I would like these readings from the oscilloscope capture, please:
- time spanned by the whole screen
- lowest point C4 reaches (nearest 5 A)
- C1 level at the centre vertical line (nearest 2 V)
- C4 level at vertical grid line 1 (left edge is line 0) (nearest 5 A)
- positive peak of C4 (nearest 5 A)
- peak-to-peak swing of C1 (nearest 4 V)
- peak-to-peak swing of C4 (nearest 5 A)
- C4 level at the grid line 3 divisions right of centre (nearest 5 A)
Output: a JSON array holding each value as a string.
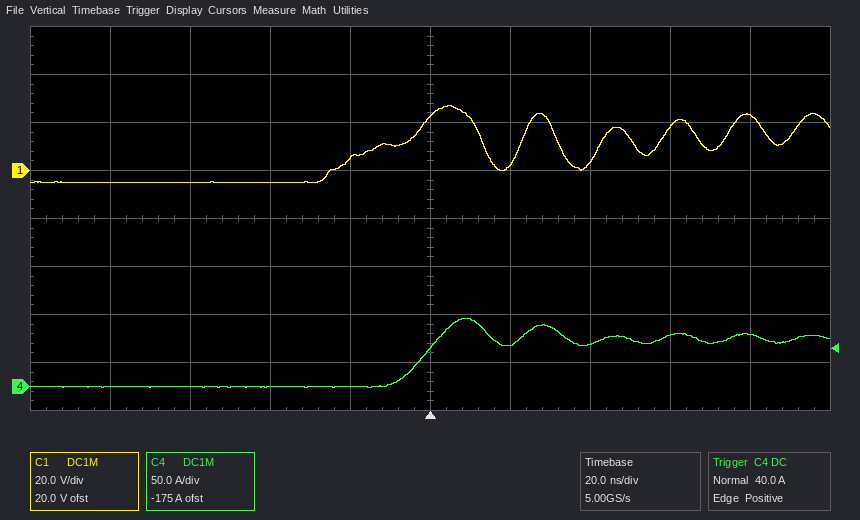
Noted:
["200 ns", "0 A", "22 V", "0 A", "70 A", "32 V", "70 A", "55 A"]
